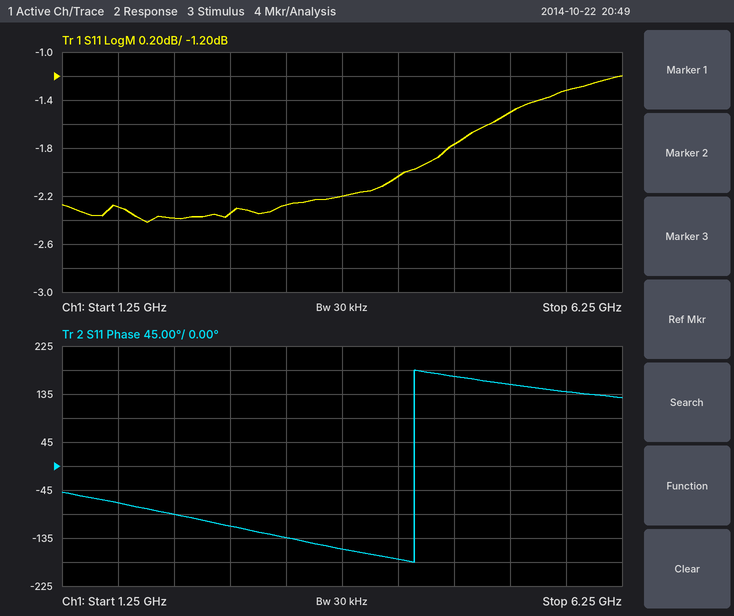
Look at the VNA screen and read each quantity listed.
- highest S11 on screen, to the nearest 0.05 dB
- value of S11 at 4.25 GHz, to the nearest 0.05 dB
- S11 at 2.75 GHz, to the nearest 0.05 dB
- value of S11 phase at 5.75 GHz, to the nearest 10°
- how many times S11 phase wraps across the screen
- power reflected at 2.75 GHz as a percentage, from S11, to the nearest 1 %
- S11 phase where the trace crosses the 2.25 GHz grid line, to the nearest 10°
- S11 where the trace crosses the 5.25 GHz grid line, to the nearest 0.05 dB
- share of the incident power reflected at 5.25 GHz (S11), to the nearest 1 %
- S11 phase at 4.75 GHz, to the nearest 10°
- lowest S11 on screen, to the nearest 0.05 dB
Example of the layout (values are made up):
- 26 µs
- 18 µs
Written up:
- -1.20 dB
- -2.05 dB
- -2.35 dB
- 140°
- 1
- 58 %
- -90°
- -1.50 dB
- 71 %
- 170°
- -2.40 dB
